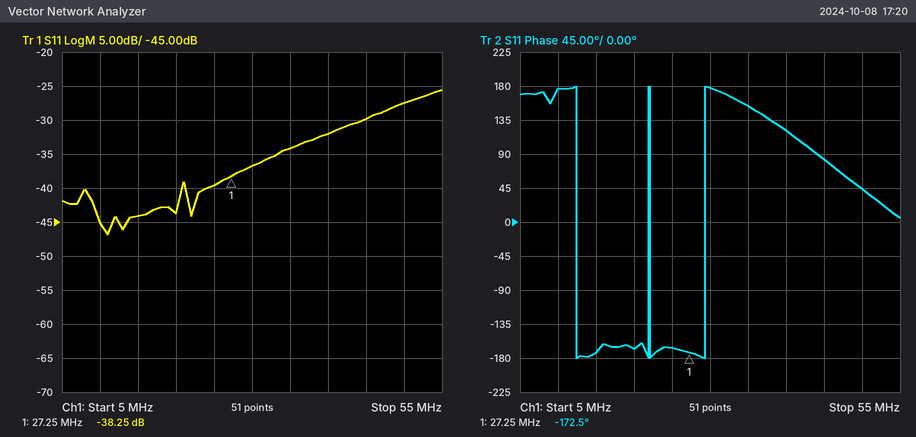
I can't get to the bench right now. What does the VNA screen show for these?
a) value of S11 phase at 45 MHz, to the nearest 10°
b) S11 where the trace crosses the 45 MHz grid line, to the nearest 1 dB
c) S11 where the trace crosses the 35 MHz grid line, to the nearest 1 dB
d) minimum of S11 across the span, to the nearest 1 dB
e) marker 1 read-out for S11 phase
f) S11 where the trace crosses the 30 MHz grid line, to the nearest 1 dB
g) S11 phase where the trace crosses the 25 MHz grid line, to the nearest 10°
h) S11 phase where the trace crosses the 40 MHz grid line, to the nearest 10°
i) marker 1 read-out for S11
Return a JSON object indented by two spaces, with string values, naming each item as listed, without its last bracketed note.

{
  "value of S11 phase at 45 MHz, to the nearest 10°": "80°",
  "S11 where the trace crosses the 45 MHz grid line, to the nearest 1 dB": "-30 dB",
  "S11 where the trace crosses the 35 MHz grid line, to the nearest 1 dB": "-34 dB",
  "minimum of S11 across the span, to the nearest 1 dB": "-47 dB",
  "marker 1 read-out for S11 phase": "-172.5°",
  "S11 where the trace crosses the 30 MHz grid line, to the nearest 1 dB": "-37 dB",
  "S11 phase where the trace crosses the 25 MHz grid line, to the nearest 10°": "-170°",
  "S11 phase where the trace crosses the 40 MHz grid line, to the nearest 10°": "120°",
  "marker 1 read-out for S11": "-38.25 dB"
}
